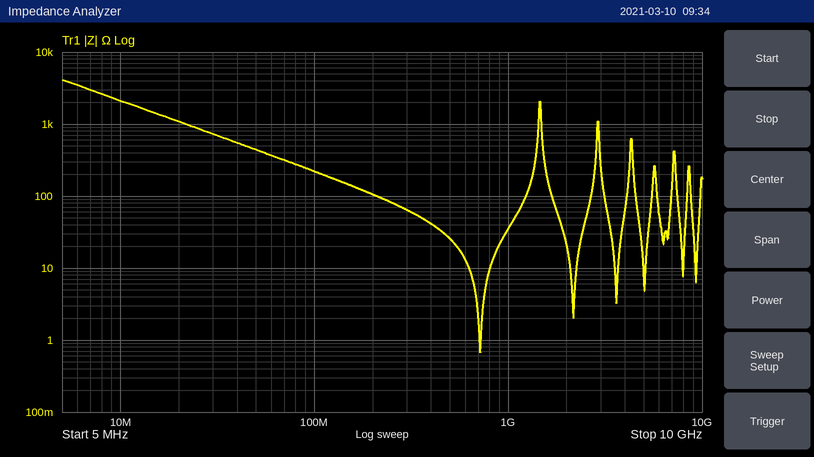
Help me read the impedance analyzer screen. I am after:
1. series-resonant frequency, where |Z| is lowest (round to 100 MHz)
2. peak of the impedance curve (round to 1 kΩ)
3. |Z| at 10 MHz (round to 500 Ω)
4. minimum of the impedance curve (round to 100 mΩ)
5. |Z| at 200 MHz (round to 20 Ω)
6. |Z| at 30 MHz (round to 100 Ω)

700 MHz
4 kΩ
2.0 kΩ
700 mΩ
100 Ω
700 Ω
